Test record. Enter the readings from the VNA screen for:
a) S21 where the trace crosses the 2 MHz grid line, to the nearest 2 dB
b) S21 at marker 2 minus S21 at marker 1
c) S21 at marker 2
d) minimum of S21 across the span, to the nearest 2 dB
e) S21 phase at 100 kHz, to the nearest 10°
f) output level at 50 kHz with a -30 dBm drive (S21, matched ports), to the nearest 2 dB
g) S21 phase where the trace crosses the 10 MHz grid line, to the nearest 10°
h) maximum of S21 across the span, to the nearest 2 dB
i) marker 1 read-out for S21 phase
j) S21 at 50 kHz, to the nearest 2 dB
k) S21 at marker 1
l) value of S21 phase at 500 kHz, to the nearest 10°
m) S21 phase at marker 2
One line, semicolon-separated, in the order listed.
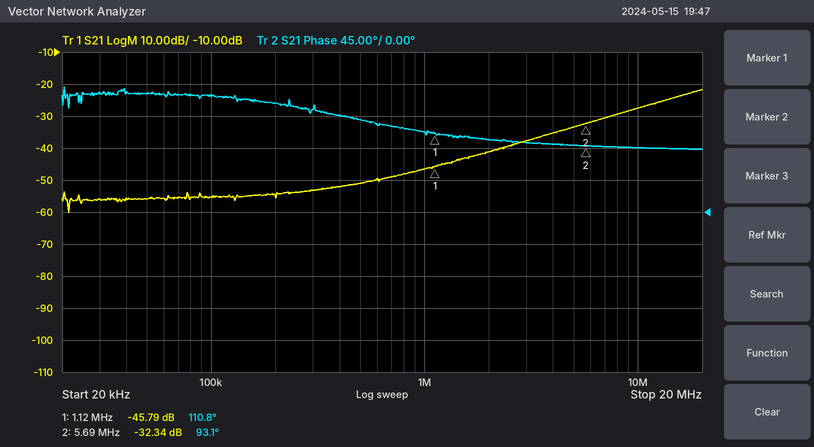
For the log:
-42 dB; 13.45 dB; -32.34 dB; -60 dB; 160°; -86 dBm; 90°; -22 dB; 110.8°; -56 dB; -45.79 dB; 130°; 93.1°
